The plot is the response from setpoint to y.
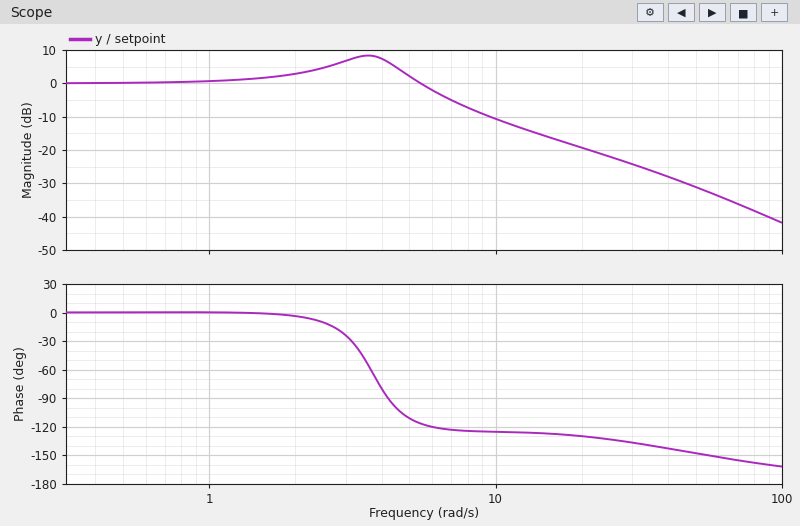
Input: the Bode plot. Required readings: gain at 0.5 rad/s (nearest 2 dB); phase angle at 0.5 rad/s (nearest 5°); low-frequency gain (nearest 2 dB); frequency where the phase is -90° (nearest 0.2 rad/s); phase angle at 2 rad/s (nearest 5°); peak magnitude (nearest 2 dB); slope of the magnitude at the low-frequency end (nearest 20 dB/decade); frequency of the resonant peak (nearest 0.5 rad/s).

0 dB
0°
0 dB
4.2 rad/s
-5°
8 dB
0 dB/decade
3.5 rad/s
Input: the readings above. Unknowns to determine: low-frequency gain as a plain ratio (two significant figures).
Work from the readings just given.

1.0
